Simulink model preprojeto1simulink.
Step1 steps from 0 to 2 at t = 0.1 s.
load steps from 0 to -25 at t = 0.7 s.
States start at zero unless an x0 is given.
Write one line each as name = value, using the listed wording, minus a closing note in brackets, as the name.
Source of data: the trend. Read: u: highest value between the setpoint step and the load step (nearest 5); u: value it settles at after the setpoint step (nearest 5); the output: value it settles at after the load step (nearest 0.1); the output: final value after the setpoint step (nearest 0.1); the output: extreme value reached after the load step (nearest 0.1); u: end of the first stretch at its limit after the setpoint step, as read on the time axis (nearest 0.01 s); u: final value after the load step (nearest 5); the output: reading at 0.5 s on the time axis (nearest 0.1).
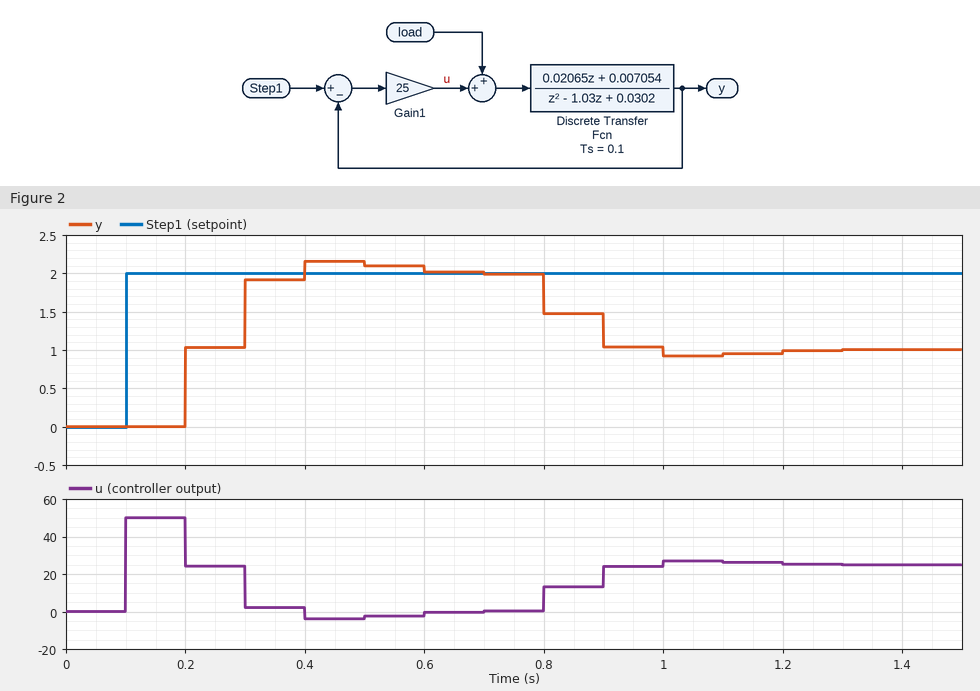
u: highest value between the setpoint step and the load step = 50
u: value it settles at after the setpoint step = 0
the output: value it settles at after the load step = 1.0
the output: final value after the setpoint step = 2.0
the output: extreme value reached after the load step = 0.9
u: end of the first stretch at its limit after the setpoint step, as read on the time axis = 0.20 s
u: final value after the load step = 25
the output: reading at 0.5 s on the time axis = 2.1
